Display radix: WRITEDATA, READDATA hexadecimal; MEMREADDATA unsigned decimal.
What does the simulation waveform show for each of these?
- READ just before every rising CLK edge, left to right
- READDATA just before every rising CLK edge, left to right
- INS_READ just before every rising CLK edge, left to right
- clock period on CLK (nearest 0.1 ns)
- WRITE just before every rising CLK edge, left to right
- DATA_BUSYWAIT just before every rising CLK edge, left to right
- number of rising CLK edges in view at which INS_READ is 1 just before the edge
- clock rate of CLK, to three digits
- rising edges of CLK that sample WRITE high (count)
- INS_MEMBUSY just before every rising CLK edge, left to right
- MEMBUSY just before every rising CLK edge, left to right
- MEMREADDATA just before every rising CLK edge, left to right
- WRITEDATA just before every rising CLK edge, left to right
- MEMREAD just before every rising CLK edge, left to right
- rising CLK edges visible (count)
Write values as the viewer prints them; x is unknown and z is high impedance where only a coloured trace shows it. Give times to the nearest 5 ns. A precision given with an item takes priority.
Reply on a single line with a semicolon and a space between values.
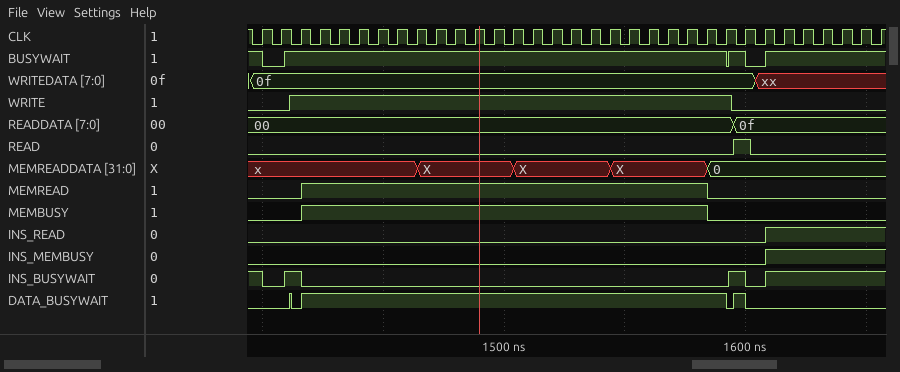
0 0 0 0 0 0 0 0 0 0 0 0 0 0 0 0 0 0 0 0 0 0 0 0 0 1 0 0 0 0 0 0 0; 00, 00, 00, 00, 00, 00, 00, 00, 00, 00, 00, 00, 00, 00, 00, 00, 00, 00, 00, 00, 00, 00, 00, 00, 00, 0f, 0f, 0f, 0f, 0f, 0f, 0f, 0f; 0 0 0 0 0 0 0 0 0 0 0 0 0 0 0 0 0 0 0 0 0 0 0 0 0 0 0 1 1 1 1 1 1; 8 ns; 0 0 1 1 1 1 1 1 1 1 1 1 1 1 1 1 1 1 1 1 1 1 1 1 1 0 0 0 0 0 0 0 0; 0 0 0 1 1 1 1 1 1 1 1 1 1 1 1 1 1 1 1 1 1 1 1 1 1 1 0 0 0 0 0 0 0; 6; 125 MHz; 23; 0 0 0 0 0 0 0 0 0 0 0 0 0 0 0 0 0 0 0 0 0 0 0 0 0 0 0 1 1 1 1 1 1; 0 0 0 1 1 1 1 1 1 1 1 1 1 1 1 1 1 1 1 1 1 1 1 1 0 0 0 0 0 0 0 0 0; x, x, x, x, x, x, x, x, x, X, X, X, X, X, X, X, X, X, X, X, X, X, X, X, 0, 0, 0, 0, 0, 0, 0, 0, 0; 0f, 0f, 0f, 0f, 0f, 0f, 0f, 0f, 0f, 0f, 0f, 0f, 0f, 0f, 0f, 0f, 0f, 0f, 0f, 0f, 0f, 0f, 0f, 0f, 0f, 0f, xx, xx, xx, xx, xx, xx, xx; 0 0 0 1 1 1 1 1 1 1 1 1 1 1 1 1 1 1 1 1 1 1 1 1 0 0 0 0 0 0 0 0 0; 33
